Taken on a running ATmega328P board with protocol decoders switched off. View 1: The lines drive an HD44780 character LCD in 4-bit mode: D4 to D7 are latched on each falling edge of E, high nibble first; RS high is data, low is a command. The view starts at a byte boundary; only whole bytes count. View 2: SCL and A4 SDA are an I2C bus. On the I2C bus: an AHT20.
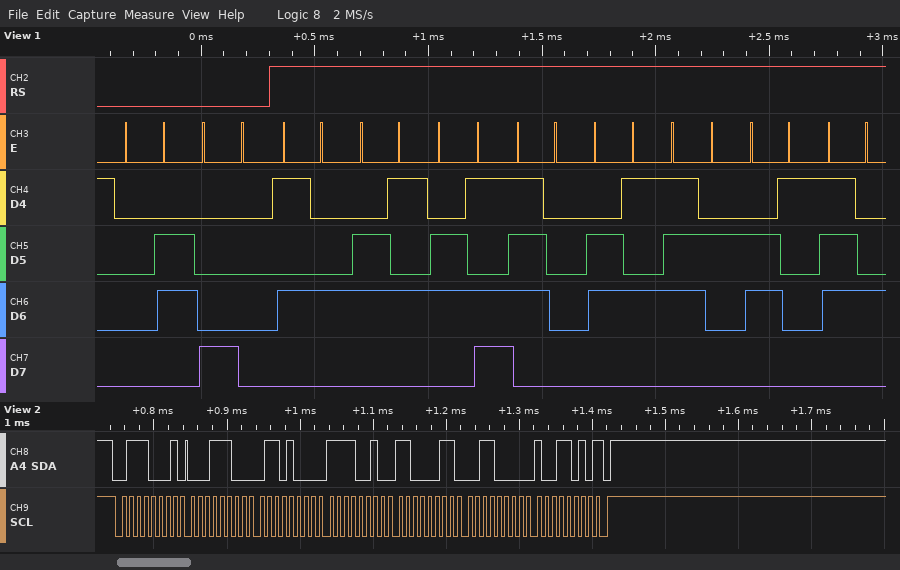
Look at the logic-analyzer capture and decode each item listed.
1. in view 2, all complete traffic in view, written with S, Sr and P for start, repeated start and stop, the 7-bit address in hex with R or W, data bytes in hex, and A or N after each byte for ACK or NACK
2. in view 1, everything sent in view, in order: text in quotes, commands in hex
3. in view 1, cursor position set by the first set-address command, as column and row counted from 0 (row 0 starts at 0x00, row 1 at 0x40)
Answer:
S 38R A 1C A 68 A F2 A C3 A 30 A 9A N P
0x06 0x80 "Temperat"
column 0, row 0
